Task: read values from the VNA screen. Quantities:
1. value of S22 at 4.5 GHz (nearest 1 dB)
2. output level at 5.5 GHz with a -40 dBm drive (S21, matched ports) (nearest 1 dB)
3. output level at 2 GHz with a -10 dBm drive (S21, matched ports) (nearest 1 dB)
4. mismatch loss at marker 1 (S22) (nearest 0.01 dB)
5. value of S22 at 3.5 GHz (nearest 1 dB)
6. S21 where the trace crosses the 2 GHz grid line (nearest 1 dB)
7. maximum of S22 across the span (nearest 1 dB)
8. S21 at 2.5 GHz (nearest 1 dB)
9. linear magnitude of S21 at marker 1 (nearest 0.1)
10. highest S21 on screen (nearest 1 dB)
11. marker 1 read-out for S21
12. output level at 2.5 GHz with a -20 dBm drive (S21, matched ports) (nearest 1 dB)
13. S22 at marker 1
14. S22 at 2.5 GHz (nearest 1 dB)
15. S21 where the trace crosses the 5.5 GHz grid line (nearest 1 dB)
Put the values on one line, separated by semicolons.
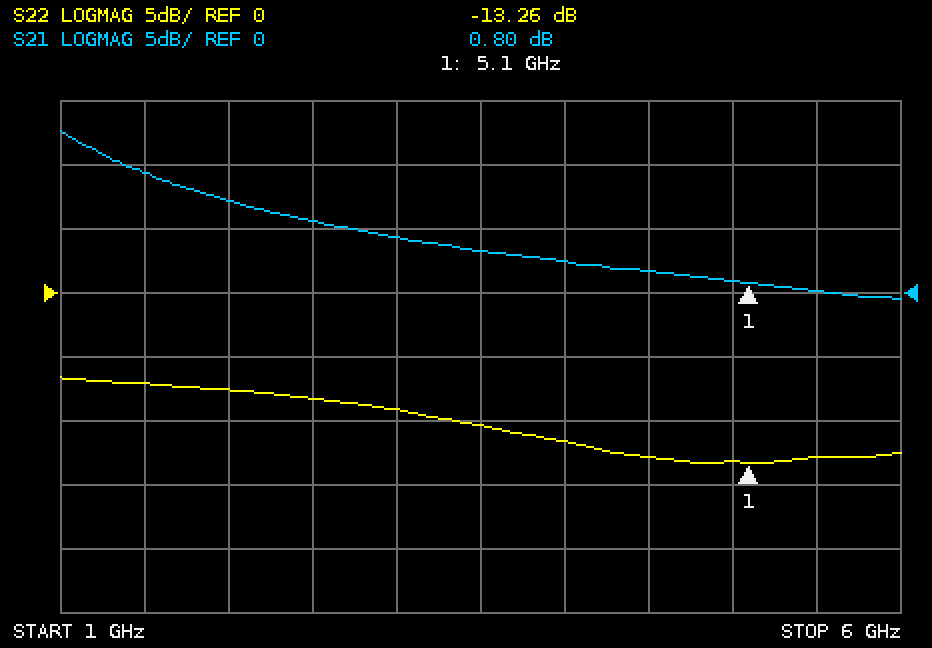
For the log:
-13 dB; -40 dBm; -3 dBm; 0.21 dB; -10 dB; 7 dB; -7 dB; 6 dB; 1.1; 13 dB; 0.80 dB; -14 dBm; -13.26 dB; -8 dB; 0 dB
